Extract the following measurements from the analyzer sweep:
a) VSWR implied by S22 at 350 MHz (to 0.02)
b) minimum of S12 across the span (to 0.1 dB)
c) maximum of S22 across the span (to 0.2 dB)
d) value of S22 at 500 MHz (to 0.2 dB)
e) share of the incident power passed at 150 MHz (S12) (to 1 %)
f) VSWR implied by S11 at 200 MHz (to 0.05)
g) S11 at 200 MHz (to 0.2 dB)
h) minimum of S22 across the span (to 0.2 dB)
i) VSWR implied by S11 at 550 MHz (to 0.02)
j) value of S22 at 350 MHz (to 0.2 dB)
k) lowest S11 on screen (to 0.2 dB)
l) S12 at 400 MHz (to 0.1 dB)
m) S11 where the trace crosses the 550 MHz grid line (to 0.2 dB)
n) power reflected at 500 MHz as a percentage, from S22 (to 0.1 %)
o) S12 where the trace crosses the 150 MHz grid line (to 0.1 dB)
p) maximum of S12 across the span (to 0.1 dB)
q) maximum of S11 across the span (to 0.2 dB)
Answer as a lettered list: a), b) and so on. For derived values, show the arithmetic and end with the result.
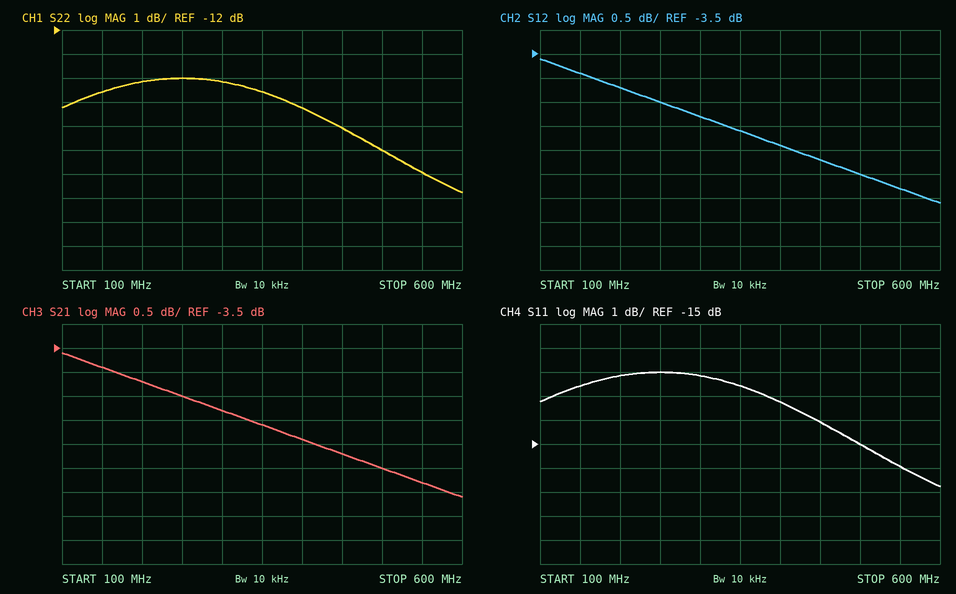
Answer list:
a) |Γ| = 10^(-14.6/20) = 0.1862; VSWR = (1 + 0.1862)/(1 − 0.1862) ≈ 1.46
b) -6.6 dB
c) -14.0 dB
d) -17.0 dB
e) 10^(-3.9/10) ≈ 41 %
f) |Γ| = 10^(-12.2/20) = 0.2455; VSWR = (1 + 0.2455)/(1 − 0.2455) ≈ 1.65
g) -12.2 dB
h) -18.8 dB
i) |Γ| = 10^(-16/20) = 0.1585; VSWR = (1 + 0.1585)/(1 − 0.1585) ≈ 1.38
j) -14.6 dB
k) -16.8 dB
l) -5.4 dB
m) -16.0 dB
n) 10^(-17/10) ≈ 2.0 %
o) -3.9 dB
p) -3.6 dB
q) -12.0 dB
